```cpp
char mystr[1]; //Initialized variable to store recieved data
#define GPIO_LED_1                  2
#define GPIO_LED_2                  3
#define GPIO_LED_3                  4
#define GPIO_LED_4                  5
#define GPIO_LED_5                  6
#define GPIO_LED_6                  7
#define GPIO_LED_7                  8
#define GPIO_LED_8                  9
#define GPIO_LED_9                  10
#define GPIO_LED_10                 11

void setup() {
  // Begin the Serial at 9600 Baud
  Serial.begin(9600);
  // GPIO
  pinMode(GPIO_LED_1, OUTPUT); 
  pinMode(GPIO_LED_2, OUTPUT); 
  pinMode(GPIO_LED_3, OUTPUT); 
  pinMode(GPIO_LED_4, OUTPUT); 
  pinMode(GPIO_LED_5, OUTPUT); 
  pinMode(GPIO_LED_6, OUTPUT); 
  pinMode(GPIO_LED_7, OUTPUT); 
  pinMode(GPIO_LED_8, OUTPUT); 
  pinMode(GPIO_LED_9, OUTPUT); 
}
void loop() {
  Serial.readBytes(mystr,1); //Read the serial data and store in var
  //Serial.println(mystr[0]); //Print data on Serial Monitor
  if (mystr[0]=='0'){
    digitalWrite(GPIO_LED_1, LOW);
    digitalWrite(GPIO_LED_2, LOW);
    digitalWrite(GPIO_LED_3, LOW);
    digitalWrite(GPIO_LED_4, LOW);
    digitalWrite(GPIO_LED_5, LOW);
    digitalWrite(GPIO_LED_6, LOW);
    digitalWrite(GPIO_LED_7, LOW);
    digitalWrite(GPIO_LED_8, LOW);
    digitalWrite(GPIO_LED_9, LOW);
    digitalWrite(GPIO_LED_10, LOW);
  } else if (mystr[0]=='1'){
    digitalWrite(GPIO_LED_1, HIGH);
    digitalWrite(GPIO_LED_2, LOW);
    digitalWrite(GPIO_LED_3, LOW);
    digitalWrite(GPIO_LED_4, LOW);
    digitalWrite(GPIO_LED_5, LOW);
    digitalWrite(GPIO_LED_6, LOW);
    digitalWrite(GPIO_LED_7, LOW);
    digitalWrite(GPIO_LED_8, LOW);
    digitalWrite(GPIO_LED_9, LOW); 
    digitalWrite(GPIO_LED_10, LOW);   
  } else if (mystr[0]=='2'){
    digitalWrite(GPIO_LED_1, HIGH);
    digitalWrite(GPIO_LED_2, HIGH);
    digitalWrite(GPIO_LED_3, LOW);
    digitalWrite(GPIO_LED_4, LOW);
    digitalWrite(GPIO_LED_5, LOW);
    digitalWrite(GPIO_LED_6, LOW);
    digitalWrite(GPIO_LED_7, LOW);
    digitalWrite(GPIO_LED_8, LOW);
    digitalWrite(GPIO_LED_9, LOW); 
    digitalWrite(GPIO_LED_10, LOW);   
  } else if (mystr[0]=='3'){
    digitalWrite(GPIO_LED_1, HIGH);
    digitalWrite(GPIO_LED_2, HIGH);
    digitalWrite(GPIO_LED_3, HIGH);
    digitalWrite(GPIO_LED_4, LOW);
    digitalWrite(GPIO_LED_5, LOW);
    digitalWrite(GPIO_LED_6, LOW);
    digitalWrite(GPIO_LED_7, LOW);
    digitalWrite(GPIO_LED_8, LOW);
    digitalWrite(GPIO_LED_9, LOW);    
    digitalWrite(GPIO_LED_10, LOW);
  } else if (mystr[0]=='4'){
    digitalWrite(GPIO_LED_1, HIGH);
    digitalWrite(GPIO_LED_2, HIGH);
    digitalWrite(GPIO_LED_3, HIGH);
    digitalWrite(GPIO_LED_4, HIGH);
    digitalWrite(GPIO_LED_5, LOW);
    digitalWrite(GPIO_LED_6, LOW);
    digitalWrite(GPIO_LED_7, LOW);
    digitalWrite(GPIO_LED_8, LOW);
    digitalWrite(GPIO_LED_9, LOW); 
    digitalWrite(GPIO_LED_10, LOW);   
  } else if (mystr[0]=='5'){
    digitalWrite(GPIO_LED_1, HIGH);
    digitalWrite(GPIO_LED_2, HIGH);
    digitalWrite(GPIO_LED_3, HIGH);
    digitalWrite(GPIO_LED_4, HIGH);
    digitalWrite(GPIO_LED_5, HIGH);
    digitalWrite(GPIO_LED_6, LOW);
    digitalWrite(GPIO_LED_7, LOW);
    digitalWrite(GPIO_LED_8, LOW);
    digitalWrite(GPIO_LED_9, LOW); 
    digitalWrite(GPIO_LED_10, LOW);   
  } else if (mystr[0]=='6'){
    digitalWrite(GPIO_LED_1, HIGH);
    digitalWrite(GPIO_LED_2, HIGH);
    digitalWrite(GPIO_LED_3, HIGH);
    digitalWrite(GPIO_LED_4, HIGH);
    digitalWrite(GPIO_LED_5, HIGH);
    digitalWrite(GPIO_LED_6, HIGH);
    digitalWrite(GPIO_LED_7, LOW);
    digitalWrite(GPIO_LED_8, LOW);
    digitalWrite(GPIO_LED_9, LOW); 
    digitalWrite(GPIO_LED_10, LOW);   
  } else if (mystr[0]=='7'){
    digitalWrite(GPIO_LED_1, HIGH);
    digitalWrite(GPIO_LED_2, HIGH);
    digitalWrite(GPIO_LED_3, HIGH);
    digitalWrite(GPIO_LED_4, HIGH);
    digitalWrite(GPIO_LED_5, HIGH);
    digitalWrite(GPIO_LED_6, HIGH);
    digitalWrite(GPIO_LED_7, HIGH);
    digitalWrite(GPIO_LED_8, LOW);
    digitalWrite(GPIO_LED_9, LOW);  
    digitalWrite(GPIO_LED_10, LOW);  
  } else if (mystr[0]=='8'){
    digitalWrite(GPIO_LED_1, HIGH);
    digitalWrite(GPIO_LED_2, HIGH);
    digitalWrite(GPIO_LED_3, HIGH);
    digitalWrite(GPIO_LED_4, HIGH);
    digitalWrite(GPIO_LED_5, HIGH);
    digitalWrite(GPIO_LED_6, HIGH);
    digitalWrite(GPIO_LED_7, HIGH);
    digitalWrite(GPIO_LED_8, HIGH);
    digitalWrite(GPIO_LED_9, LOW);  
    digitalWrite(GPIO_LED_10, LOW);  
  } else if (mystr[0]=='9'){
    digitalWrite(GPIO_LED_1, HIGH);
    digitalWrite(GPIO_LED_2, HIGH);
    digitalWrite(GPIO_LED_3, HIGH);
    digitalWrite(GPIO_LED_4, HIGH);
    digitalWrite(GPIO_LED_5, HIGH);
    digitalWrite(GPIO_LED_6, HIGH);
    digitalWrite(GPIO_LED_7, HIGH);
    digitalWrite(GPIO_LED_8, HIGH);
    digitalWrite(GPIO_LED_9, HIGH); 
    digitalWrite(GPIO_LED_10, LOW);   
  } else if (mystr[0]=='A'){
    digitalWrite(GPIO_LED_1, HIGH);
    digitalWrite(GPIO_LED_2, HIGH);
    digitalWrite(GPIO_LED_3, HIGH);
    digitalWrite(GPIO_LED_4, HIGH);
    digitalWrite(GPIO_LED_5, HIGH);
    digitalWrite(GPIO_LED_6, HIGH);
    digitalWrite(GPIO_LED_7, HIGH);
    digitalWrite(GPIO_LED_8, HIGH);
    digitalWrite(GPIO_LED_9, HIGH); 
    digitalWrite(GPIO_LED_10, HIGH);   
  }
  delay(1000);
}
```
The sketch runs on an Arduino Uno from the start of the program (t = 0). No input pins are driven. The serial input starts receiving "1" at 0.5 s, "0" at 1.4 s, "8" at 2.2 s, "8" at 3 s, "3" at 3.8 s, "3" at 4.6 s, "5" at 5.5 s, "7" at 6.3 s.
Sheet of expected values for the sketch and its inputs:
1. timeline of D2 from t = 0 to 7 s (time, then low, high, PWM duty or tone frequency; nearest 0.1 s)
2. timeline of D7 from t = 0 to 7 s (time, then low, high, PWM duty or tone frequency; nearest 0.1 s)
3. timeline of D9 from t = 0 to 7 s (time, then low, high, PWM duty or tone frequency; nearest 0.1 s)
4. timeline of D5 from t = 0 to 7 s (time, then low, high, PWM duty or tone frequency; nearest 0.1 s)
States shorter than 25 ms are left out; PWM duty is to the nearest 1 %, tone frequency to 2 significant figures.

0 s low; 0.5 s high; 1.5 s low; 2.5 s high
0 s low; 2.5 s high; 4.5 s low
0 s low; 2.5 s high; 4.5 s low
0 s low; 2.5 s high; 4.5 s low; 6.5 s high
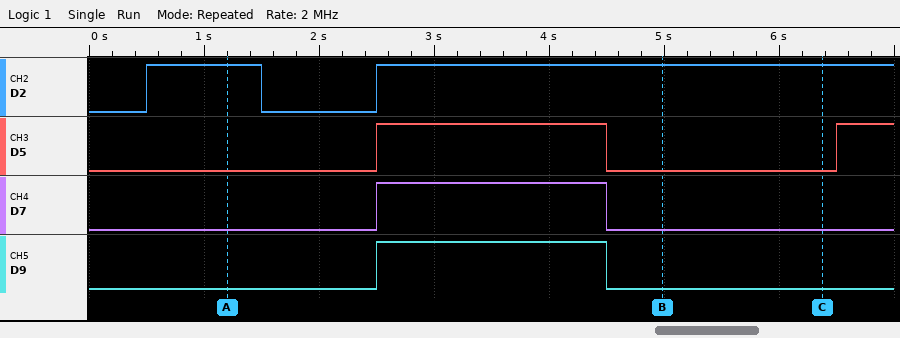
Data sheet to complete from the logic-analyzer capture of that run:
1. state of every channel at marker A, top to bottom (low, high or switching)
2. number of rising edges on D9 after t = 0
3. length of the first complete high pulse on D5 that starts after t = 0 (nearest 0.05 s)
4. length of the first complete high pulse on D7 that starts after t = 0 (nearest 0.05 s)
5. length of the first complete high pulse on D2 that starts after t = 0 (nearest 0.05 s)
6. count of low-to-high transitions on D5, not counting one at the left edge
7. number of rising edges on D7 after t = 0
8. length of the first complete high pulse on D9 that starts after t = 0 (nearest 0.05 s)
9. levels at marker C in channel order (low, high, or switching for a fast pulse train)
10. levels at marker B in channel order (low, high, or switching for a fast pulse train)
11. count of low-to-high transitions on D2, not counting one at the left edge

D2 high, D5 low, D7 low, D9 low
1
2.00 s
2.00 s
1.00 s
2
1
2.00 s
D2 high, D5 low, D7 low, D9 low
D2 high, D5 low, D7 low, D9 low
2
